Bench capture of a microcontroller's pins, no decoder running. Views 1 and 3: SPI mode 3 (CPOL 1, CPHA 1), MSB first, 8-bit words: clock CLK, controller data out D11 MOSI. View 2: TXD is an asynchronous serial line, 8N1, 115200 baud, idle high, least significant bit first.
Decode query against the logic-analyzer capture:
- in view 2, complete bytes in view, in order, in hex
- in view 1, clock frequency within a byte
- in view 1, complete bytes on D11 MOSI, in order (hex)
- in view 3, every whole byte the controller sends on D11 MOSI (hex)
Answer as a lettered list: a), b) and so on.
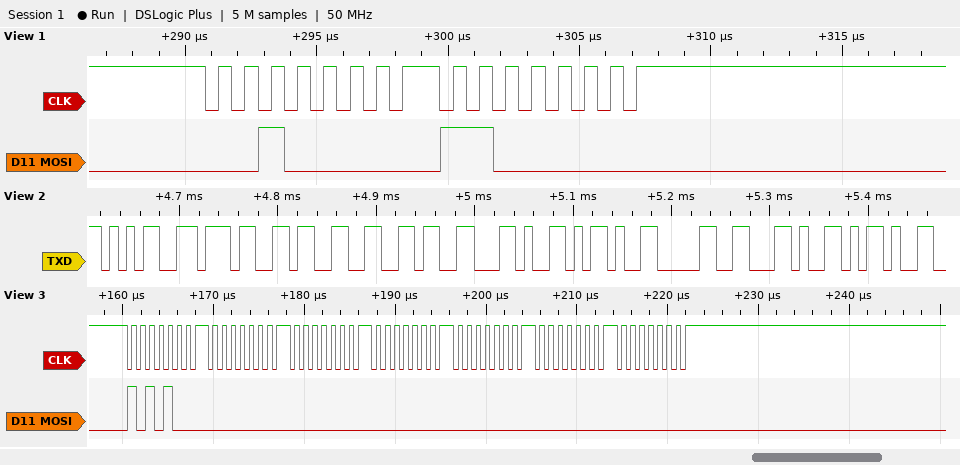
a) 35 37 33 36 2C 2D 30 2C 2D
b) 1 MHz
c) 20 C0
d) A8 00 00 00 00 00 00
